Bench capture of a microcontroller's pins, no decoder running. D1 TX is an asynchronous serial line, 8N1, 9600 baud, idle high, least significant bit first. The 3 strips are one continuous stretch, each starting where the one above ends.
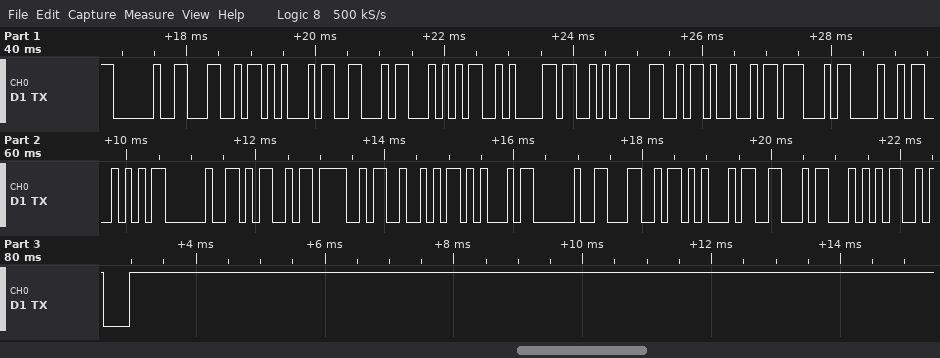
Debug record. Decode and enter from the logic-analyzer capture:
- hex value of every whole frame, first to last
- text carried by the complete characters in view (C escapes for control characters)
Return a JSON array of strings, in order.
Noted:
["20 4C 45 46 54 0A 53 4C 49 47 48 54 20 4D 4F 52 45 20 4C 45 46 54 0A", "\" LEFT\\nSLIGHT MORE LEFT\\n\""]
